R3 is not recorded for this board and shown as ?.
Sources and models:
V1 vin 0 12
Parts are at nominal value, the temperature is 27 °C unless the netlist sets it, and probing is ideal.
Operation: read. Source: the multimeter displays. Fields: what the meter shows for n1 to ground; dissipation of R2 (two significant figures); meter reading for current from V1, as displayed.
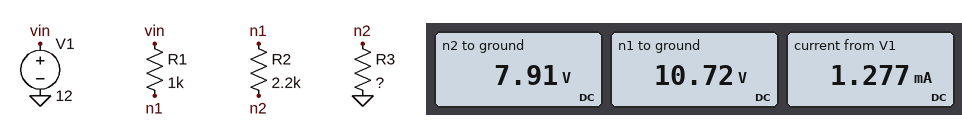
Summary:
10.72 V
3.6 mW
1.277 mA
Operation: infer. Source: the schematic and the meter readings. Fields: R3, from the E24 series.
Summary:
6.2 kΩ
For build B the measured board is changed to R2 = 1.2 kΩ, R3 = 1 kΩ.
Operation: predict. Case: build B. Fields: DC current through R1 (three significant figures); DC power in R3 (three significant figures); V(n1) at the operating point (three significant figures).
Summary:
3.75 mA
14.1 mW
8.25 V
